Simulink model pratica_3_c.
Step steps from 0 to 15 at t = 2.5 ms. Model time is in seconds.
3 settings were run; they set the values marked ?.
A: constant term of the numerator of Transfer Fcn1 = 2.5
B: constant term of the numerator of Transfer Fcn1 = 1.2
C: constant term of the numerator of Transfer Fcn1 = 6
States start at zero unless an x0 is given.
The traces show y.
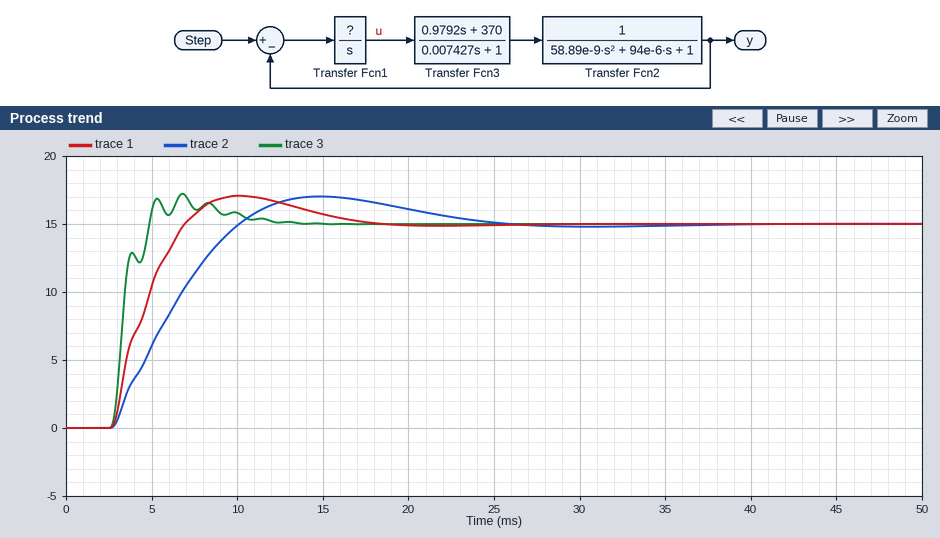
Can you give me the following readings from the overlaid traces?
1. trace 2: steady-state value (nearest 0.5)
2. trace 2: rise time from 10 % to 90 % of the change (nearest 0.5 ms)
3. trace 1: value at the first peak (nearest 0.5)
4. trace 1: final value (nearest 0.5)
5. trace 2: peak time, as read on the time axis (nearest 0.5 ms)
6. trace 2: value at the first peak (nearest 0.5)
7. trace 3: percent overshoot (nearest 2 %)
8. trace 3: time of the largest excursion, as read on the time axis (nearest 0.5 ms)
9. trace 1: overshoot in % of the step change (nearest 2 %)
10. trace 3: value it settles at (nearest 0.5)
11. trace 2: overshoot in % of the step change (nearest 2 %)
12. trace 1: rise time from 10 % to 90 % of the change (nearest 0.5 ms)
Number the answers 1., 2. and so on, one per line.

1. 15.0
2. 5.5 ms
3. 17.0
4. 15.0
5. 15.0 ms
6. 17.0
7. 14 %
8. 7.0 ms
9. 14 %
10. 15.0
11. 14 %
12. 3.0 ms
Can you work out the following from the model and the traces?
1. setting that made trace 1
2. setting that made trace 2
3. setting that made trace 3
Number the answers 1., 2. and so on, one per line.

1. A
2. B
3. C
